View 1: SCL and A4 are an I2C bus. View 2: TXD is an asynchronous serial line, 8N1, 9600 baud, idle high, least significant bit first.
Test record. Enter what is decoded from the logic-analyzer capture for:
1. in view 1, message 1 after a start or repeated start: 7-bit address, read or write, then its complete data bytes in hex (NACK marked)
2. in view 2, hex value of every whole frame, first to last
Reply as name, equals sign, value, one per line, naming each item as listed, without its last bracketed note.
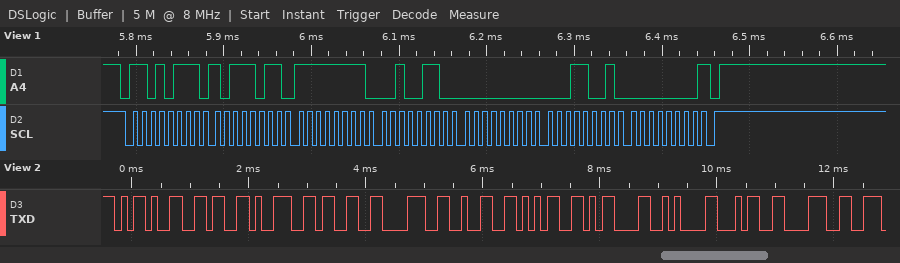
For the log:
in view 1, message 1 after a start or repeated start: 7-bit address, read or write, then its complete data bytes in hex = 0x6B read: BB FF 26 00 19 00 NACK
in view 2, hex value of every whole frame, first to last = 2D 36 39 33 38 32 35 0D 0A 34 38
